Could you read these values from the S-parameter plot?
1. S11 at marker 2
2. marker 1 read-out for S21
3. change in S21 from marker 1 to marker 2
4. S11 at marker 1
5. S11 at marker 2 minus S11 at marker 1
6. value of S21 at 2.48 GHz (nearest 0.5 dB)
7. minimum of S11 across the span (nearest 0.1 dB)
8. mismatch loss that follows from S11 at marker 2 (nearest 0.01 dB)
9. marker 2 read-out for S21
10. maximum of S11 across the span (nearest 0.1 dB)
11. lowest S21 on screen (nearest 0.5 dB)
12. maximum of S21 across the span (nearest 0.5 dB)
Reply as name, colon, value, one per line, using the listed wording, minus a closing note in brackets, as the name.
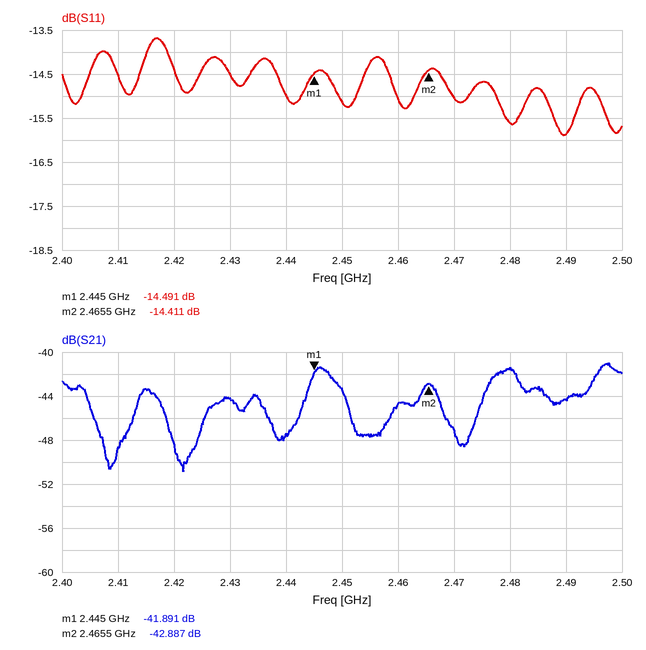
S11 at marker 2: -14.411 dB
marker 1 read-out for S21: -41.891 dB
change in S21 from marker 1 to marker 2: -0.996 dB
S11 at marker 1: -14.491 dB
S11 at marker 2 minus S11 at marker 1: 0.080 dB
value of S21 at 2.48 GHz: -41.5 dB
minimum of S11 across the span: -15.9 dB
mismatch loss that follows from S11 at marker 2: 0.16 dB
marker 2 read-out for S21: -42.887 dB
maximum of S11 across the span: -13.7 dB
lowest S21 on screen: -51.0 dB
maximum of S21 across the span: -41.0 dB
